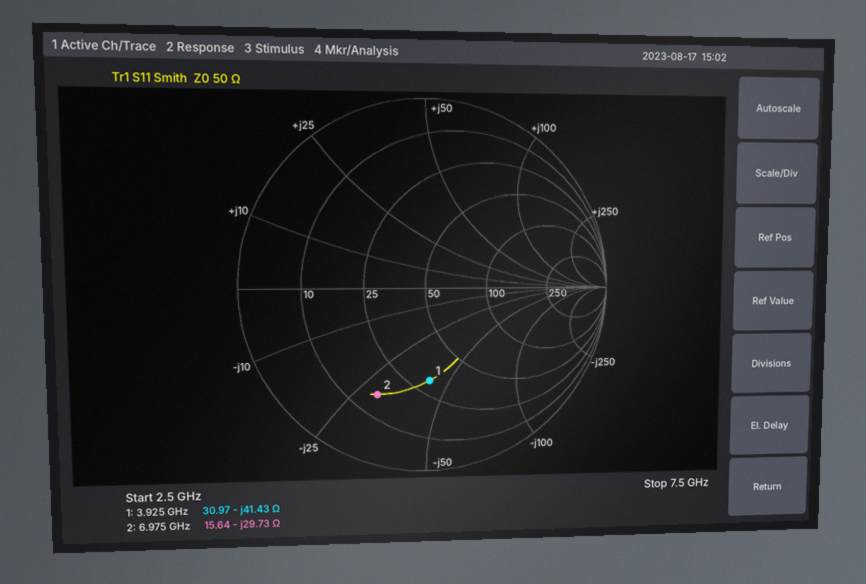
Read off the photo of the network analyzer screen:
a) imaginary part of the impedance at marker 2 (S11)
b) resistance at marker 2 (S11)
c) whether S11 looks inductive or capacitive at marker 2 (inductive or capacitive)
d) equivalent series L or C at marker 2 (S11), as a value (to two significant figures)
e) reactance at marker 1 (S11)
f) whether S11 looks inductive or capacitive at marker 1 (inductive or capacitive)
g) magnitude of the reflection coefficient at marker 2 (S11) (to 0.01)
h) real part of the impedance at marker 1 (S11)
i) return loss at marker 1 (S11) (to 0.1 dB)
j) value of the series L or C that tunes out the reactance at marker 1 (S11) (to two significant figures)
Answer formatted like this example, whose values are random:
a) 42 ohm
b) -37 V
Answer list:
a) -29.73 Ω
b) 15.64 Ω
c) capacitive
d) 770 fF
e) -41.43 Ω
f) capacitive
g) 0.63
h) 30.97 Ω
i) 6.0 dB
j) 1.7 nH
